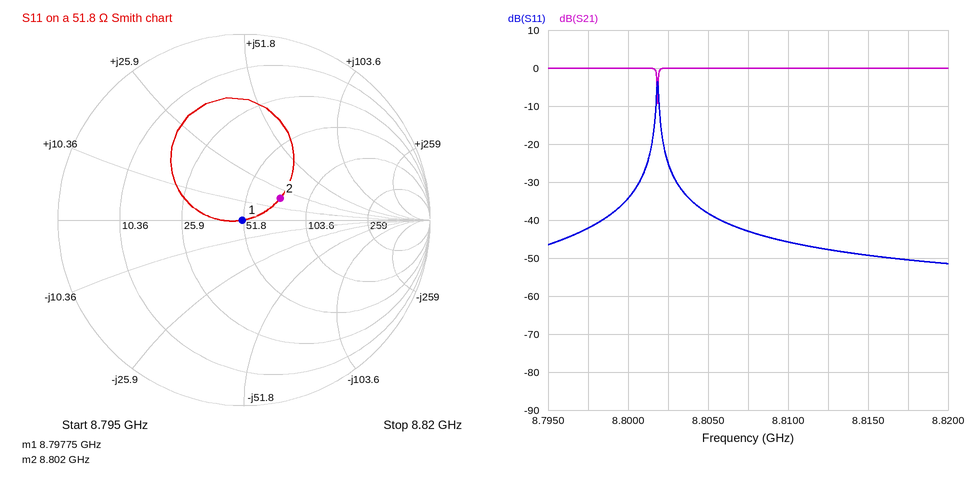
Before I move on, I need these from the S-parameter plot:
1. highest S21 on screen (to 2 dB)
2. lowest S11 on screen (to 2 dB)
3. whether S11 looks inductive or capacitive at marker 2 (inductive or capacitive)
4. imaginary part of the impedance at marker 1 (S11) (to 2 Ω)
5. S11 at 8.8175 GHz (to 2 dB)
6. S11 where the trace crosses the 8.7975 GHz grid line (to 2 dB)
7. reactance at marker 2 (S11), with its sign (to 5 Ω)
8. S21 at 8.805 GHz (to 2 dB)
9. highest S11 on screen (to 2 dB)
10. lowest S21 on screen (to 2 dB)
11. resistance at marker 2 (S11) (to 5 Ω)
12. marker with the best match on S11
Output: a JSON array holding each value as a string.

["0 dB", "-52 dB", "inductive", "0 Ω", "-50 dB", "-42 dB", "+20 Ω", "0 dB", "-4 dB", "-10 dB", "75 Ω", "marker 1"]
